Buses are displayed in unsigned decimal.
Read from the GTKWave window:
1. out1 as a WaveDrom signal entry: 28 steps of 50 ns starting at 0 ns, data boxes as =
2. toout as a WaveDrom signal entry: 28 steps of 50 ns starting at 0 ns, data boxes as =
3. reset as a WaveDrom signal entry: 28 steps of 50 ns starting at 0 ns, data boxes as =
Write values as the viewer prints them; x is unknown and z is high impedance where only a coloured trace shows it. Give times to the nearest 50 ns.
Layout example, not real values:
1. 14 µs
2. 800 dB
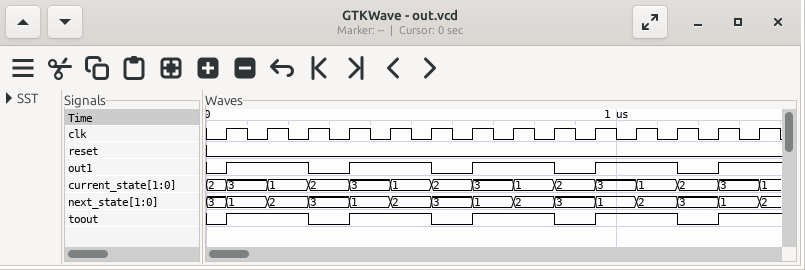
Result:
1. {name: 'out1', wave: '01...0.1...0.1...0.1...0.1..'}
2. {name: 'toout', wave: '01...0.1...0.1...0.1...0.1..'}
3. {name: 'reset', wave: '0...........................'}
